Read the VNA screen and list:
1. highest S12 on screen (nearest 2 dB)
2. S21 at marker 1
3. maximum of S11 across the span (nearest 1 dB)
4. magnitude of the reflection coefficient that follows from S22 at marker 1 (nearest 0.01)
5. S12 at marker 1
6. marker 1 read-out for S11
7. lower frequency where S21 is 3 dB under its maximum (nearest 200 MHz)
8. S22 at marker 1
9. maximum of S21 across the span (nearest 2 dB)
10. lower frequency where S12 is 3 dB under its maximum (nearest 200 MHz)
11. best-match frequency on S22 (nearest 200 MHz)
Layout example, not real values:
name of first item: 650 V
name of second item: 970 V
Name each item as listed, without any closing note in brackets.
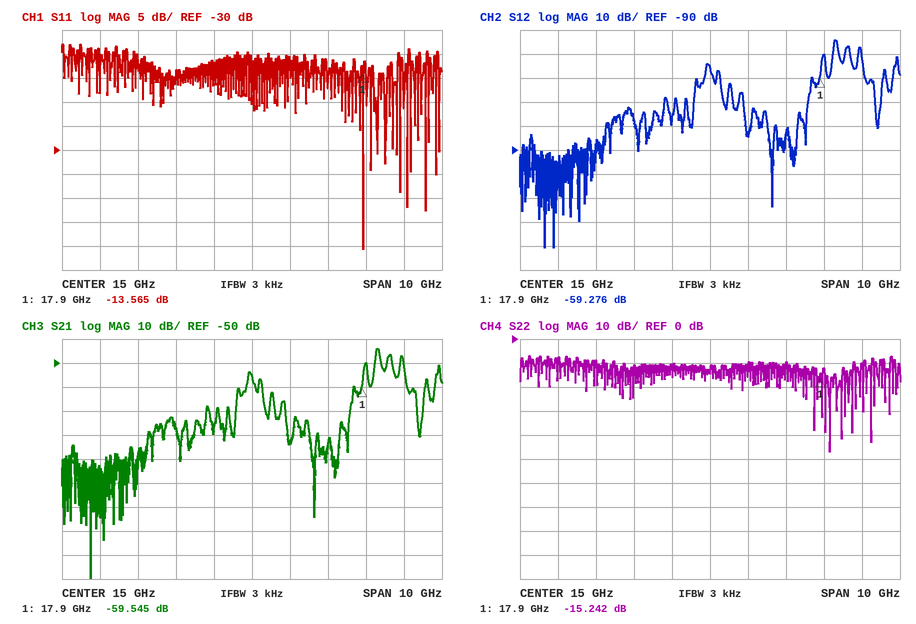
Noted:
highest S12 on screen: -44 dB
S21 at marker 1: -59.545 dB
maximum of S11 across the span: -8 dB
magnitude of the reflection coefficient that follows from S22 at marker 1: 0.17
S12 at marker 1: -59.276 dB
marker 1 read-out for S11: -13.565 dB
lower frequency where S21 is 3 dB under its maximum: 18.2 GHz
S22 at marker 1: -15.242 dB
maximum of S21 across the span: -44 dB
lower frequency where S12 is 3 dB under its maximum: 18.2 GHz
best-match frequency on S22: 18.2 GHz
